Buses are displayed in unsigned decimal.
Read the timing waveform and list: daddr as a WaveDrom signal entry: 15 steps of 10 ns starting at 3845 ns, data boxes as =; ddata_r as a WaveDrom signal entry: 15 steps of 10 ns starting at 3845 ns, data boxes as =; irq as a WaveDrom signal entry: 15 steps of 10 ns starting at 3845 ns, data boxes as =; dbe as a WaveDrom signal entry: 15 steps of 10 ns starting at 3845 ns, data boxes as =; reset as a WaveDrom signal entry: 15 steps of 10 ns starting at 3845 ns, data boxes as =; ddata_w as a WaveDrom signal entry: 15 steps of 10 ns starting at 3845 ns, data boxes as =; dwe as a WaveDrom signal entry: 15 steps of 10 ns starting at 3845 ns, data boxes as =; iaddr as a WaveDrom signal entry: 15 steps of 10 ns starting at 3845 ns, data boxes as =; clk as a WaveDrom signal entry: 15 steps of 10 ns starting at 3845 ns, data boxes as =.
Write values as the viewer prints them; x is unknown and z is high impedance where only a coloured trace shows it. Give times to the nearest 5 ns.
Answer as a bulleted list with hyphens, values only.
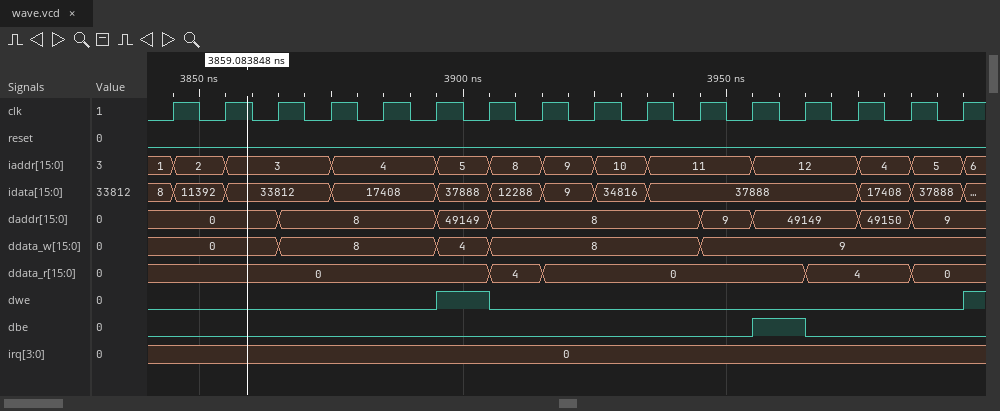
- {name: 'daddr', wave: '=.=..==...==.==', data: '0 8 49149 8 9 49149 49150 9'}
- {name: 'ddata_r', wave: '=.....==....=.=', data: '0 4 0 4 0'}
- {name: 'irq', wave: '=..............', data: '0'}
- {name: 'dbe', wave: '0..........10..'}
- {name: 'reset', wave: '0..............'}
- {name: 'ddata_w', wave: '=.=..==...=....', data: '0 8 4 8 9'}
- {name: 'dwe', wave: '0....10........'}
- {name: 'iaddr', wave: '==.=.=====.=.==', data: '2 3 4 5 8 9 10 11 12 4 5'}
- {name: 'clk', wave: 'p..............'}
